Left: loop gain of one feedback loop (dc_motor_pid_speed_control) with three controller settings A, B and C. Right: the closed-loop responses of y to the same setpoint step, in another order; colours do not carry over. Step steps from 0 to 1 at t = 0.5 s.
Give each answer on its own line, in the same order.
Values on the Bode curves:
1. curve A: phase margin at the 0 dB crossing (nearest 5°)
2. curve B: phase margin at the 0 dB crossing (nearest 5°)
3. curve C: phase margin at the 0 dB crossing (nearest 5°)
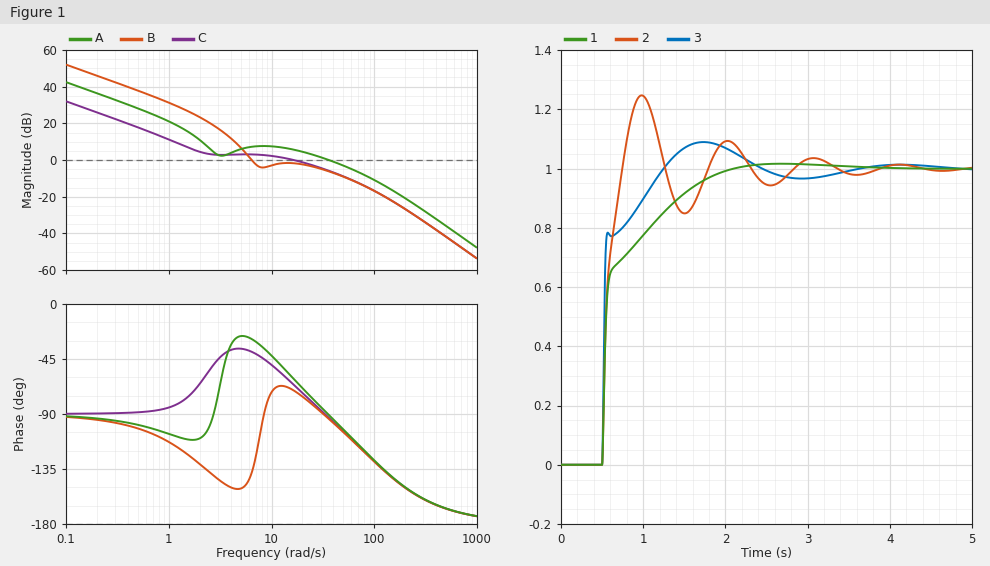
90°
40°
115°
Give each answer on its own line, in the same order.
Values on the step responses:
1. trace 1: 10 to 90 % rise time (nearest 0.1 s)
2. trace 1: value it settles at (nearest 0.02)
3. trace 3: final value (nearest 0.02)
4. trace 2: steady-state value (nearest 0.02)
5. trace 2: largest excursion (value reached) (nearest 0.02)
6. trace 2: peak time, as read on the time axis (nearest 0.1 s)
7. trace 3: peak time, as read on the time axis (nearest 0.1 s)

0.9 s
1.00
1.00
1.00
1.24
1.0 s
1.7 s
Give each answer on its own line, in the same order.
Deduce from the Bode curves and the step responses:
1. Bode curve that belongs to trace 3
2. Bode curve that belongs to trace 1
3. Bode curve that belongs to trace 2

A
C
B
